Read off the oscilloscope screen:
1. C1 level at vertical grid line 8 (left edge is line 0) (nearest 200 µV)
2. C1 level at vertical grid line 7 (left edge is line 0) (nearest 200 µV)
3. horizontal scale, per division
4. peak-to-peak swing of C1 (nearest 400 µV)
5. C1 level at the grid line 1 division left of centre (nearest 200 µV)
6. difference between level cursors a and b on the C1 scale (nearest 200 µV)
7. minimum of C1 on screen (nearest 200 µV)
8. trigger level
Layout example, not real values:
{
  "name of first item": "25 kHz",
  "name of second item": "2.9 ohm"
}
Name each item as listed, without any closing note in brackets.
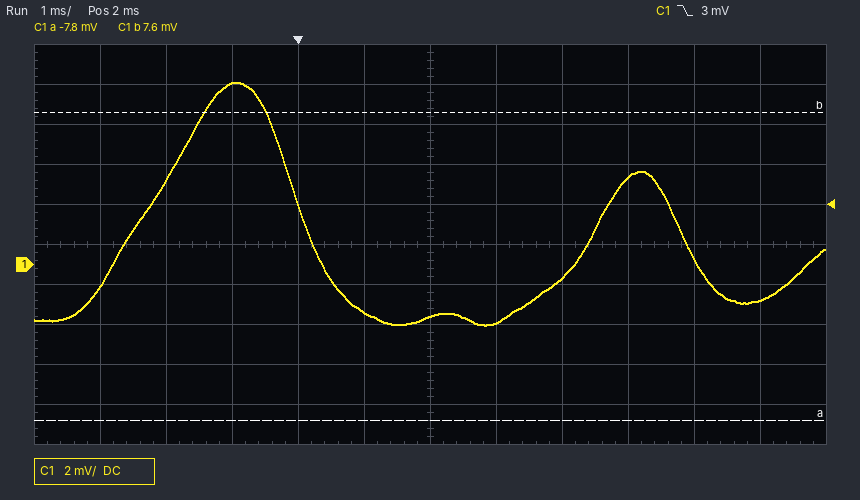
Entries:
{
  "C1 level at vertical grid line 8 (left edge is line 0)": "-600 µV",
  "C1 level at vertical grid line 7 (left edge is line 0)": "-3.0 mV",
  "horizontal scale, per division": "1 ms",
  "peak-to-peak swing of C1": "12.0 mV",
  "C1 level at the grid line 1 division left of centre": "-2.4 mV",
  "difference between level cursors a and b on the C1 scale": "15.4 mV",
  "minimum of C1 on screen": "-3.0 mV",
  "trigger level": "3 mV"
}
